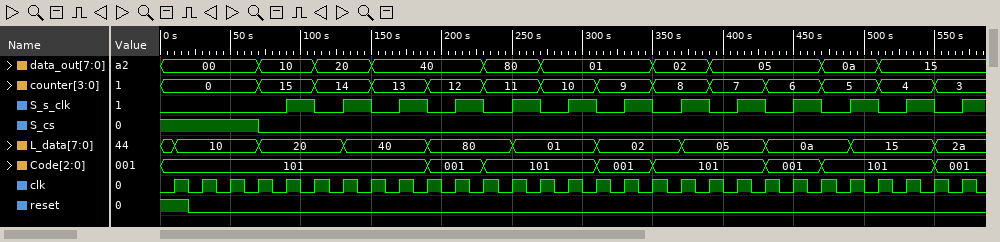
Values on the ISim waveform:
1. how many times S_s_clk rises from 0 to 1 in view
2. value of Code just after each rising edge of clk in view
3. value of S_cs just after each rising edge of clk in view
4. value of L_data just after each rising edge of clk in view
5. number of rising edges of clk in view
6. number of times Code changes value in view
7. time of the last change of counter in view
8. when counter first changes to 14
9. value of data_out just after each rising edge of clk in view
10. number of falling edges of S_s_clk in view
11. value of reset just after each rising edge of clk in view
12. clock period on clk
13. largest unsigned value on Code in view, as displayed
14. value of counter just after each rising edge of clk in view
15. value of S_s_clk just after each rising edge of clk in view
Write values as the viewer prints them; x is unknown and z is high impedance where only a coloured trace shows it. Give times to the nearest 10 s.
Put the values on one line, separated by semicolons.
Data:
13; 101, 101, 101, 101, 101, 101, 101, 101, 101, 001, 001, 101, 101, 101, 101, 001, 001, 101, 101, 101, 101, 001, 001, 101, 101, 101, 101, 001, 001; 1 1 1 0 0 0 0 0 0 0 0 0 0 0 0 0 0 0 0 0 0 0 0 0 0 0 0 0 0; 10, 10, 10, 20, 20, 20, 40, 40, 40, 80, 80, 80, 01, 01, 01, 02, 02, 02, 05, 05, 05, 0a, 0a, 0a, 15, 15, 15, 2a, 2a; 29; 7; 550 s; 110 s; 00, 00, 00, 10, 10, 20, 20, 40, 40, 40, 40, 80, 80, 01, 01, 01, 01, 02, 02, 05, 05, 05, 05, 0a, 0a, 15, 15, 15, 15; 12; 1 0 0 0 0 0 0 0 0 0 0 0 0 0 0 0 0 0 0 0 0 0 0 0 0 0 0 0 0; 20 s; 101; 0, 0, 0, 15, 15, 14, 14, 13, 13, 12, 12, 11, 11, 10, 10, 9, 9, 8, 8, 7, 7, 6, 6, 5, 5, 4, 4, 3, 3; 0 0 0 0 1 0 1 0 1 0 1 0 1 0 1 0 1 0 1 0 1 0 1 0 1 0 1 0 1
